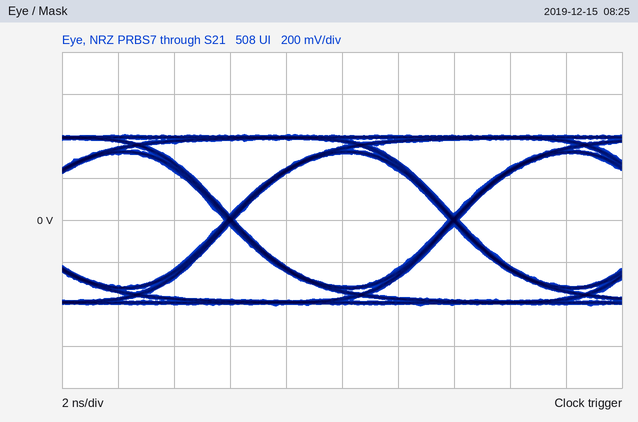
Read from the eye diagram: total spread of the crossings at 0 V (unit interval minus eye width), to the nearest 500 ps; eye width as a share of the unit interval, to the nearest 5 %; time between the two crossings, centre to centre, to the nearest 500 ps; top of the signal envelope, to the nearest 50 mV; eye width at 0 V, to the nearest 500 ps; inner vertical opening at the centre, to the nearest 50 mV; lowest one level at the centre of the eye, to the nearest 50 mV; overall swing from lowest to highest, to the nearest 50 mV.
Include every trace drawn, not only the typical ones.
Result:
500 ps
95 %
8.0 ns
400 mV
7.5 ns
650 mV
300 mV
800 mV
